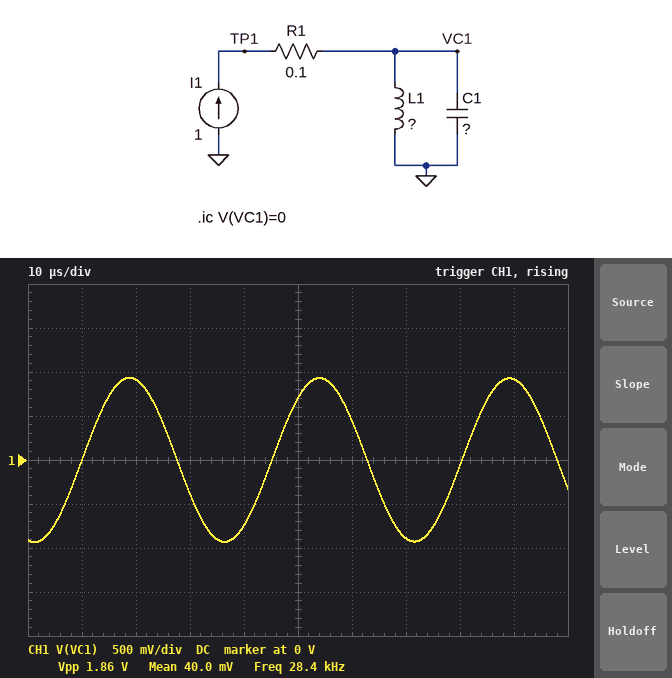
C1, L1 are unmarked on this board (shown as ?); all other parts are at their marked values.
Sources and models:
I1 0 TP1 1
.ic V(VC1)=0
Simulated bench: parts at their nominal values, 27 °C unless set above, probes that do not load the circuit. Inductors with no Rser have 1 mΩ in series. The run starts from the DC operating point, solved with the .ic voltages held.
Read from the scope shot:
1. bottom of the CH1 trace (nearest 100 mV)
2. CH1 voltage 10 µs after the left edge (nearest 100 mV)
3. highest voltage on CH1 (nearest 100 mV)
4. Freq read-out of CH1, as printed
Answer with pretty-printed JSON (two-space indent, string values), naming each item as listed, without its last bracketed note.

{
  "bottom of the CH1 trace": "-900 mV",
  "CH1 voltage 10 µs after the left edge": "0 V",
  "highest voltage on CH1": "900 mV",
  "Freq read-out of CH1, as printed": "28.4 kHz"
}
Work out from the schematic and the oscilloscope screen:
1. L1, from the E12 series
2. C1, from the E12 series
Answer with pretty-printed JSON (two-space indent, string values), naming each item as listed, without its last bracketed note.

{
  "L1, from the E12 series": "5.6 µH",
  "C1, from the E12 series": "5.6 µF"
}
